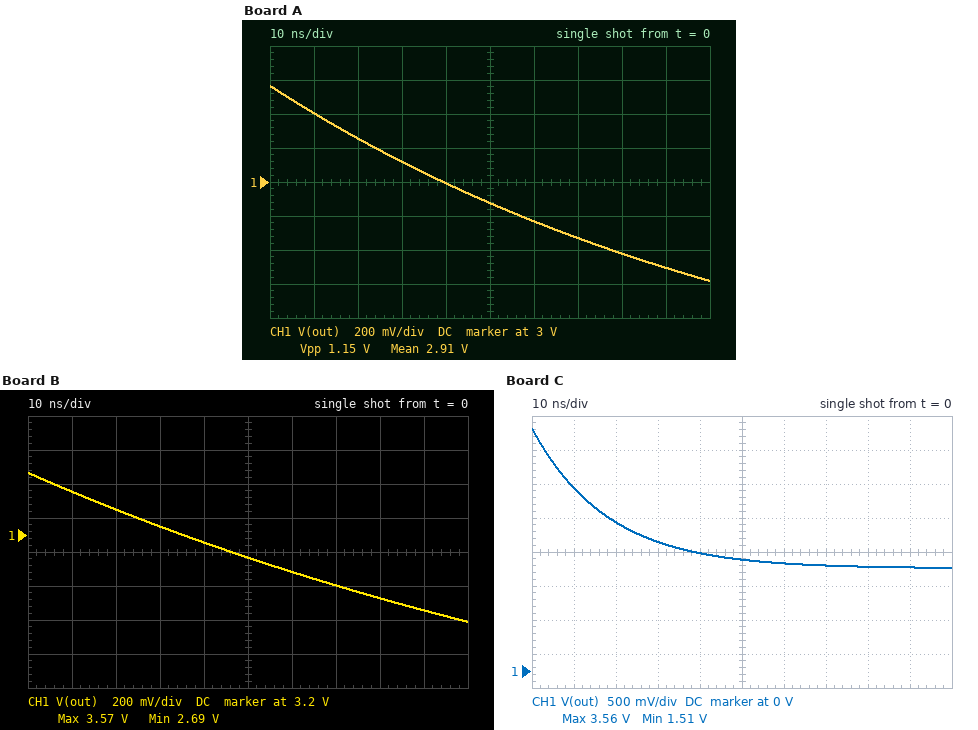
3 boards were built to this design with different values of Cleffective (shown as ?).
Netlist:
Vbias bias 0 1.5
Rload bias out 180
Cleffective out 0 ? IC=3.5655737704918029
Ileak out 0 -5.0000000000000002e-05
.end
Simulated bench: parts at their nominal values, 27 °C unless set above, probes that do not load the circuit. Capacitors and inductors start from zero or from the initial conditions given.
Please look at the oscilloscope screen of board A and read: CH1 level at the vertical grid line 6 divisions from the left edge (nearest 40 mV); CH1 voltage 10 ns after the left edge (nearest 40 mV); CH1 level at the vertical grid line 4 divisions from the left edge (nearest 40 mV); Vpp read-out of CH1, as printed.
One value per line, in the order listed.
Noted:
2.76 V
3.40 V
3.00 V
1.15 V
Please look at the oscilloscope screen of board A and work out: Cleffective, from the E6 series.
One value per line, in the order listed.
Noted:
680 pF
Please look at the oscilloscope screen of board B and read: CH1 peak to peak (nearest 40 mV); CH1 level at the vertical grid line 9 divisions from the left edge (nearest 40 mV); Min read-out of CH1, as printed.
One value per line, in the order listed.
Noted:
880 mV
2.76 V
2.69 V
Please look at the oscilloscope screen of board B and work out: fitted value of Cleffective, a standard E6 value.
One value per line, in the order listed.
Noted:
1 nF
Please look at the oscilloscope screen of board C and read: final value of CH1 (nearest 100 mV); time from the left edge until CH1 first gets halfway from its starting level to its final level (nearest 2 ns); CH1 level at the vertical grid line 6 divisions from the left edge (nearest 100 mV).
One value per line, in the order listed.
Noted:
1.5 V
12 ns
1.6 V
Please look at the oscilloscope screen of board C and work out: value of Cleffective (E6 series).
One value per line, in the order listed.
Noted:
100 pF
